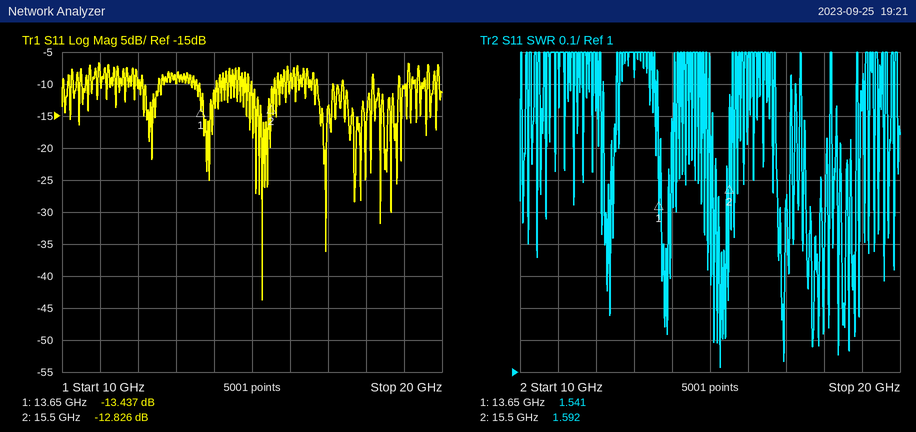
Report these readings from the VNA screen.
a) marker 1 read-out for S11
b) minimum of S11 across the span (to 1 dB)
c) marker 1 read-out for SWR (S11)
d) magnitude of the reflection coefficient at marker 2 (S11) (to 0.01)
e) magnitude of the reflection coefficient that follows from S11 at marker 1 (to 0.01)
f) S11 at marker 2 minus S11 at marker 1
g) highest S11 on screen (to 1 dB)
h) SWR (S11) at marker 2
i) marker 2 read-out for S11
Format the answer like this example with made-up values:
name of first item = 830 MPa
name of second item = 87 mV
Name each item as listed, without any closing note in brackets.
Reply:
marker 1 read-out for S11 = -13.437 dB
minimum of S11 across the span = -44 dB
marker 1 read-out for SWR = 1.541
magnitude of the reflection coefficient at marker 2 (S11) = 0.23
magnitude of the reflection coefficient that follows from S11 at marker 1 = 0.21
S11 at marker 2 minus S11 at marker 1 = 0.611 dB
highest S11 on screen = -7 dB
SWR (S11) at marker 2 = 1.592
marker 2 read-out for S11 = -12.826 dB
